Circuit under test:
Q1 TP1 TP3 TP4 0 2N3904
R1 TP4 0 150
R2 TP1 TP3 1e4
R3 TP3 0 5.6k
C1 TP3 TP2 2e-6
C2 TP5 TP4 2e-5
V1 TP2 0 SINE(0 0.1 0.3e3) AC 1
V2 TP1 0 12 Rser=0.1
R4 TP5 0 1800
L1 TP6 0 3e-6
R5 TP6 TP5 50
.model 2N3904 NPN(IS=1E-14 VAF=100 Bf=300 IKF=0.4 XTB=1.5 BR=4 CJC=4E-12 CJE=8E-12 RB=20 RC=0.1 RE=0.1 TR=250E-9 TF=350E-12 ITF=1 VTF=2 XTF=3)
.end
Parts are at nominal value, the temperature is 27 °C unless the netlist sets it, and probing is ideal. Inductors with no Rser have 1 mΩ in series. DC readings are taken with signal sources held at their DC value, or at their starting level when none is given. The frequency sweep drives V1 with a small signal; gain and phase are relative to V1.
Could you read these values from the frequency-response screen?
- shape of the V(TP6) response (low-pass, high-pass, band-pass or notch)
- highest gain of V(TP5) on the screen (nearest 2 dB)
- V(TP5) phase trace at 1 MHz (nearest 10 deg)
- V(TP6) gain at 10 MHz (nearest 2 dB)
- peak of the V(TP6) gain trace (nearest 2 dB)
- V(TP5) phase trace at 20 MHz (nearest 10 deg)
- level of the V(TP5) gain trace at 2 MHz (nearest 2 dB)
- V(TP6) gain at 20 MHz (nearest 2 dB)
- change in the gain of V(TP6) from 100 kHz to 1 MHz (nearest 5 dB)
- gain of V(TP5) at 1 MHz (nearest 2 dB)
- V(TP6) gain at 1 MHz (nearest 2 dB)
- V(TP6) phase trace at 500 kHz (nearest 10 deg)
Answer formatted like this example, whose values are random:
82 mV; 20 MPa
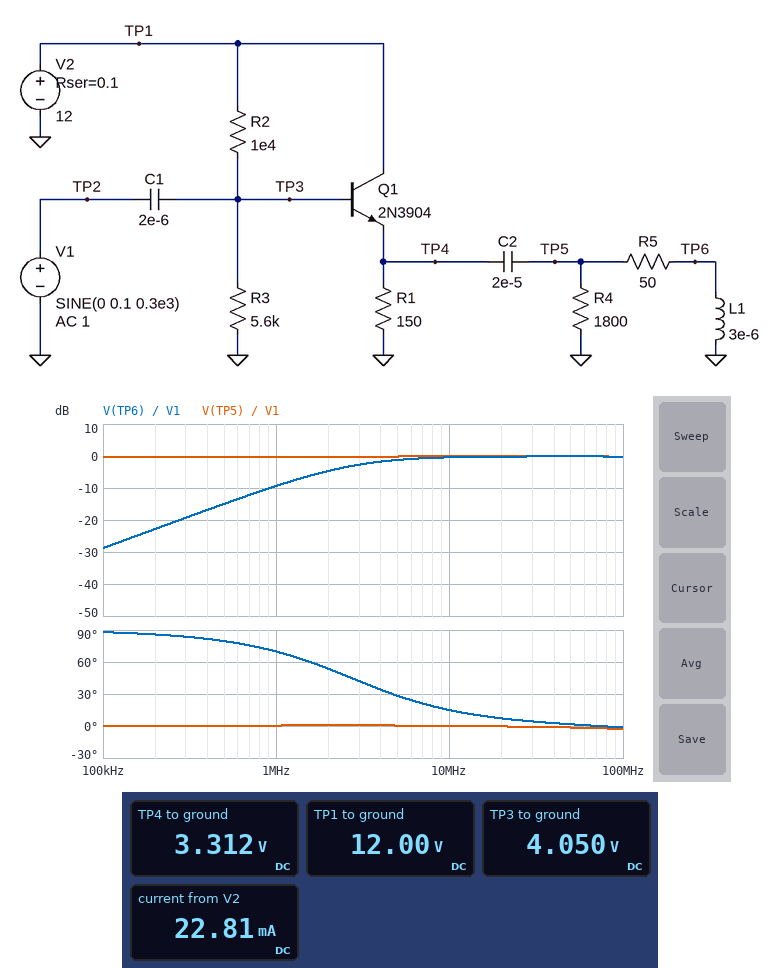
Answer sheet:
high-pass; 0 dB; 0 deg; 0 dB; 0 dB; 0 deg; 0 dB; 0 dB; 20 dB; 0 dB; -10 dB; 80 deg
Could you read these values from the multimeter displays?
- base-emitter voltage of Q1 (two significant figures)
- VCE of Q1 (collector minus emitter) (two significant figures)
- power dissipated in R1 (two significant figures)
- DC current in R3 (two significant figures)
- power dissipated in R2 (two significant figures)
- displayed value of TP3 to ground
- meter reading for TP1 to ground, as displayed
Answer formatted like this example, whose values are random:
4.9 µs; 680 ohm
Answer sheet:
740 mV; 8.7 V; 73 mW; 720 µA; 6.3 mW; 4.050 V; 12.00 V
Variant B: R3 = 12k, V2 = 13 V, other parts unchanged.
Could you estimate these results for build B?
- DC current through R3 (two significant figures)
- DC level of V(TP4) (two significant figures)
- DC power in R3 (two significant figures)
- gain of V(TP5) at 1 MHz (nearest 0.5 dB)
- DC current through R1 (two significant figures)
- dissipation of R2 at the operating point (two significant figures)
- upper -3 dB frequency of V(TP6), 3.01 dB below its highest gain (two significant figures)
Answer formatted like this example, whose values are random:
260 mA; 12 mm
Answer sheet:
530 µA; 5.6 V; 3.4 mW; 0 dB; 38 mA; 4.4 mW; 3.5 GHz
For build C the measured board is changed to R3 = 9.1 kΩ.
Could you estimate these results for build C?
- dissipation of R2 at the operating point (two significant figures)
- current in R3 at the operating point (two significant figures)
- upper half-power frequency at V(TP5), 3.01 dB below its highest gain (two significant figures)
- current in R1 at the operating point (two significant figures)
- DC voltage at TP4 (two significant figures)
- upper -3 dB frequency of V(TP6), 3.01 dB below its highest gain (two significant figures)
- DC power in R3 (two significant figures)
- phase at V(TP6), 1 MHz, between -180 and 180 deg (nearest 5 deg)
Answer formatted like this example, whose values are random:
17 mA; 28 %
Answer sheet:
4.6 mW; 580 µA; 3.5 GHz; 30 mA; 4.5 V; 3.6 GHz; 3.0 mW; 70 deg
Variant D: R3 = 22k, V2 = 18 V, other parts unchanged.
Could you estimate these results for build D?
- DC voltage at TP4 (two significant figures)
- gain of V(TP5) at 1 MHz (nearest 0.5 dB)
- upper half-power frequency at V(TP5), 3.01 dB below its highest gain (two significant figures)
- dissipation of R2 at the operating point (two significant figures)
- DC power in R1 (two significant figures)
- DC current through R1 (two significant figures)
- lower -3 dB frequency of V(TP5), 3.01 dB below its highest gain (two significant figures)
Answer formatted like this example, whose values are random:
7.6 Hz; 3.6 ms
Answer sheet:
10 V; 0 dB; 3.6 GHz; 5.3 mW; 660 mW; 66 mA; 170 Hz
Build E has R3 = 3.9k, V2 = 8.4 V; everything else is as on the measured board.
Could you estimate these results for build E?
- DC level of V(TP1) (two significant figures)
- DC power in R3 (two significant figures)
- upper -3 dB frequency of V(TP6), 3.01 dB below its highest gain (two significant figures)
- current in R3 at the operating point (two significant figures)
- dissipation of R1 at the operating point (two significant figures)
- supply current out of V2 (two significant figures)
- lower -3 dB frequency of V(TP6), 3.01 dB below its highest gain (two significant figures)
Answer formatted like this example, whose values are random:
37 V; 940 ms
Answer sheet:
8.4 V; 1.3 mW; 3.6 GHz; 580 µA; 16 mW; 11 mA; 2.8 MHz
